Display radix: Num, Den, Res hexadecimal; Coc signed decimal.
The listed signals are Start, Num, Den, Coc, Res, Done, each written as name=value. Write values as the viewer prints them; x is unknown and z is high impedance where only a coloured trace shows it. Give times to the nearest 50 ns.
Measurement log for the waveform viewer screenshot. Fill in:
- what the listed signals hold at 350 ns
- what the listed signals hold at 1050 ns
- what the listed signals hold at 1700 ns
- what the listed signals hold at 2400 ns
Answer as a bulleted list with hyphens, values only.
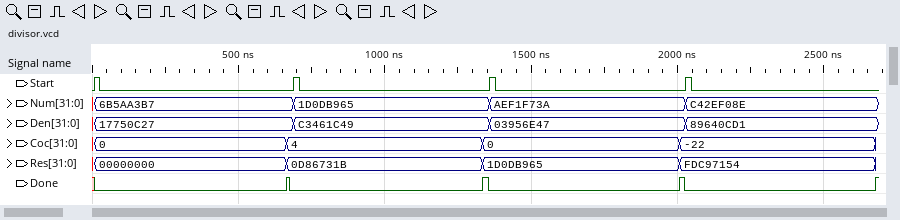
- Start=0, Num=6B5AA3B7, Den=17750C27, Coc=0, Res=00000000, Done=0
- Start=0, Num=1D0DB965, Den=C3461C49, Coc=4, Res=0D86731B, Done=0
- Start=0, Num=AEF1F73A, Den=03956E47, Coc=0, Res=1D0DB965, Done=0
- Start=0, Num=C42EF08E, Den=89640CD1, Coc=-22, Res=FDC97154, Done=0
